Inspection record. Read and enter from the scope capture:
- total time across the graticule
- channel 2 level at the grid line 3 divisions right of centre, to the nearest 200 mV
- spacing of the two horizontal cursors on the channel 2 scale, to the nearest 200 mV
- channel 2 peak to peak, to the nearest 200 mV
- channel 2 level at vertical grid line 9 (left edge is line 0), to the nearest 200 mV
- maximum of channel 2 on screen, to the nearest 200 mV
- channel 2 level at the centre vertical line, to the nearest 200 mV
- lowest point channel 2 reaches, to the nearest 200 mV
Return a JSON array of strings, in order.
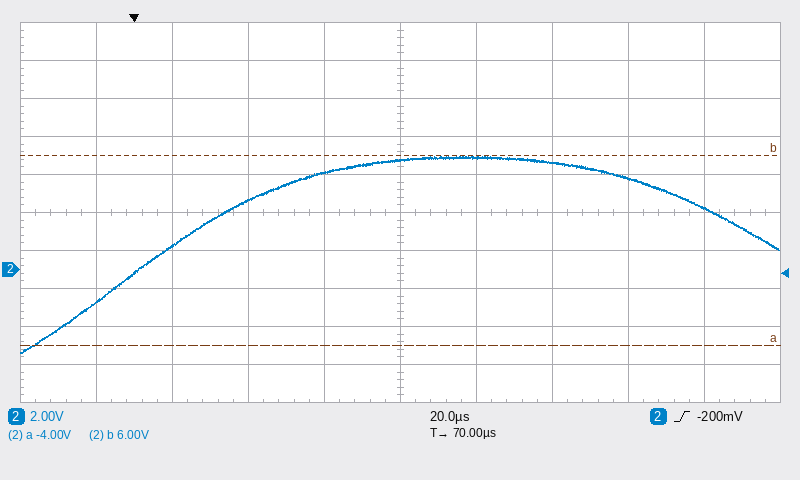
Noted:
["200 µs", "4.8 V", "10.0 V", "10.4 V", "3.2 V", "6.0 V", "5.8 V", "-4.4 V"]
